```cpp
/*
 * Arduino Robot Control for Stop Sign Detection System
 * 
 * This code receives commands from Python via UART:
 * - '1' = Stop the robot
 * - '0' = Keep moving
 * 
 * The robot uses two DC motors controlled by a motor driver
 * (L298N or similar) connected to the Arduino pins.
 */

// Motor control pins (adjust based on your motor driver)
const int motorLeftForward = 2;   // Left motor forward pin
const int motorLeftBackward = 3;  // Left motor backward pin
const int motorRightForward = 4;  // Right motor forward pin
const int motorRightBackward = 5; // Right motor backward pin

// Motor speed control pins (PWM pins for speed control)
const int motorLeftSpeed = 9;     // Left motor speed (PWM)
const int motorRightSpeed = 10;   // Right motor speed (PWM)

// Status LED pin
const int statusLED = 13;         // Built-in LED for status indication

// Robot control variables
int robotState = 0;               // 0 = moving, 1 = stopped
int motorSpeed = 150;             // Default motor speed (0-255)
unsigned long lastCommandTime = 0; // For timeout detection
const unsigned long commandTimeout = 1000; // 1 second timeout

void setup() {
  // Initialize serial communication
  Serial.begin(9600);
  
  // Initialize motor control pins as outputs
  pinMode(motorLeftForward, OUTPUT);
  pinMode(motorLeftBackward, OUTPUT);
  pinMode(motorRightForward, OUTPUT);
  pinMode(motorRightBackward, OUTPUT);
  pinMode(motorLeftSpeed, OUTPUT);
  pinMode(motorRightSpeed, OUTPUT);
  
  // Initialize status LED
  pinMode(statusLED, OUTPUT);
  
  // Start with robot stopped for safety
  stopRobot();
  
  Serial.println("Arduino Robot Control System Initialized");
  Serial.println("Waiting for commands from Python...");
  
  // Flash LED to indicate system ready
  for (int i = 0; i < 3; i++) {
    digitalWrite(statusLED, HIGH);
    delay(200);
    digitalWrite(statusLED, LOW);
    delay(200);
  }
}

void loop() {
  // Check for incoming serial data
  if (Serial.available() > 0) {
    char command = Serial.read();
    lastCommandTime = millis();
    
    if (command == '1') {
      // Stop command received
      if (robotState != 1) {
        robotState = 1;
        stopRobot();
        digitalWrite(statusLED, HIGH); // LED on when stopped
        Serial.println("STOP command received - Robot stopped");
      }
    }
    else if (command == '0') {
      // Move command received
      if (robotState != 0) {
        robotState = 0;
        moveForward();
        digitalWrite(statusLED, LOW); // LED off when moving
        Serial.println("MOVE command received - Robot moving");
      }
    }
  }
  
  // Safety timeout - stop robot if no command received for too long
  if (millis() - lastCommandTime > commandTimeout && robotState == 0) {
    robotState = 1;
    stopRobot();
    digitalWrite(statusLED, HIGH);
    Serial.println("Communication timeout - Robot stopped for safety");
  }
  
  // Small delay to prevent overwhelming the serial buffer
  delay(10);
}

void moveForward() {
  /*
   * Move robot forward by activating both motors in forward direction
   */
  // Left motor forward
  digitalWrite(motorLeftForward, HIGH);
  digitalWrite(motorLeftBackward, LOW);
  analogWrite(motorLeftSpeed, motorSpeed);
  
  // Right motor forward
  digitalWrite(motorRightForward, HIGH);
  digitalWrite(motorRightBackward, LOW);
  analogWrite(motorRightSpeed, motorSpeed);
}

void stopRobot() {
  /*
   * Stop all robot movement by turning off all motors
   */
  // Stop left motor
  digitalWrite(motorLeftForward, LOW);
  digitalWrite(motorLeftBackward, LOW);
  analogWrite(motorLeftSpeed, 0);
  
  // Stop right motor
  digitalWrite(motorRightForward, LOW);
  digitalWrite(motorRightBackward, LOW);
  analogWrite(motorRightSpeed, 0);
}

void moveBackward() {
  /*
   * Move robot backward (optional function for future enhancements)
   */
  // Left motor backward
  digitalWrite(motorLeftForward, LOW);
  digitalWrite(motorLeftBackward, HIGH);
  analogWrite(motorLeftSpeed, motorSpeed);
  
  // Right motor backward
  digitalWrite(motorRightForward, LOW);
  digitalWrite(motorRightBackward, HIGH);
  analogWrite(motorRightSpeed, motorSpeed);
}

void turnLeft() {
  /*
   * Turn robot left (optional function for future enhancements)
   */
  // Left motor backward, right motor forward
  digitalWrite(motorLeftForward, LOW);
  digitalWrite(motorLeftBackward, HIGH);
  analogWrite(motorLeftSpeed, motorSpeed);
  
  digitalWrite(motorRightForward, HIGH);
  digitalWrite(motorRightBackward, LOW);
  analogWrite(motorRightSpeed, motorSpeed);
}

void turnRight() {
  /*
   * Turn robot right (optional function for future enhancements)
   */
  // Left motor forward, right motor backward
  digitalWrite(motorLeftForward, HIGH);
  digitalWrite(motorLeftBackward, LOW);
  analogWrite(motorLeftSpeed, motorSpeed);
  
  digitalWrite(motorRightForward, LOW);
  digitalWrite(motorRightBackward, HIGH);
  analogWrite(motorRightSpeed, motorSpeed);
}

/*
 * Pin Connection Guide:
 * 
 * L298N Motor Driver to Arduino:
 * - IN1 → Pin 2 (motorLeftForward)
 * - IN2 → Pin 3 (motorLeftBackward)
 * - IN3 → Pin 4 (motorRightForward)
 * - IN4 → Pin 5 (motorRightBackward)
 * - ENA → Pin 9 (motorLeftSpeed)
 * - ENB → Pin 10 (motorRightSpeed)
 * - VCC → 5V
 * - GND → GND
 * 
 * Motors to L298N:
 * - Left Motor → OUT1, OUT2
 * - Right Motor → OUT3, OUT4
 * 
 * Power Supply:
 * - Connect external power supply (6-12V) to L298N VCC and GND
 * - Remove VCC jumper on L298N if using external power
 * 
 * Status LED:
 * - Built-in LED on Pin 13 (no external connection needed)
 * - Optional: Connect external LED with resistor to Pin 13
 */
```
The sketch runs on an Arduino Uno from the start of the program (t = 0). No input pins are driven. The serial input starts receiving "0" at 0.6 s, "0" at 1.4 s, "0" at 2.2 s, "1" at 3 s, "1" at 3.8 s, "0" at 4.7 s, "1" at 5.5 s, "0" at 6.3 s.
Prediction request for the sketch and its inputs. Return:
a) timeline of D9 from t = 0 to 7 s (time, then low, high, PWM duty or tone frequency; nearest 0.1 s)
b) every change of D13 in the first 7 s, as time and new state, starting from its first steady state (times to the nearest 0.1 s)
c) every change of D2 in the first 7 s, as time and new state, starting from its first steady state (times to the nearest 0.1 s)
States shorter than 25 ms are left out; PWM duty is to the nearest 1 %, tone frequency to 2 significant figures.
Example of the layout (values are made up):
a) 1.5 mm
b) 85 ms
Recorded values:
a) 0 s low; 4.7 s PWM 59 %; 5.5 s low; 6.3 s PWM 59 %
b) 0 s high; 0.2 s low; 0.4 s high; 0.6 s low; 0.8 s high; 1 s low; 3 s high; 4.7 s low; 5.5 s high; 6.3 s low
c) 0 s low; 4.7 s high; 5.5 s low; 6.3 s high
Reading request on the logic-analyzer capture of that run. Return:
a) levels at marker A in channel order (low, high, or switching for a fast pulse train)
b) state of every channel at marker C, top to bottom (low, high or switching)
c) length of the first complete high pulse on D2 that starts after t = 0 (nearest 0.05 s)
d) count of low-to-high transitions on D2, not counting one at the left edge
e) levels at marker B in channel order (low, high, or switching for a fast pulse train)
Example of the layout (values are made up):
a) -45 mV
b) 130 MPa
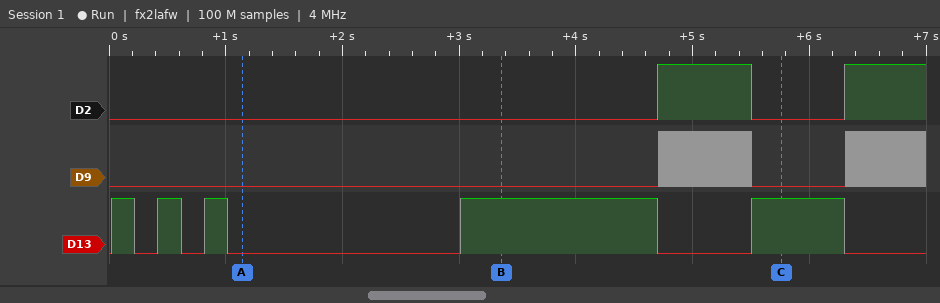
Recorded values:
a) D2 low, D9 low, D13 low
b) D2 low, D9 low, D13 high
c) 0.80 s
d) 2
e) D2 low, D9 low, D13 high
